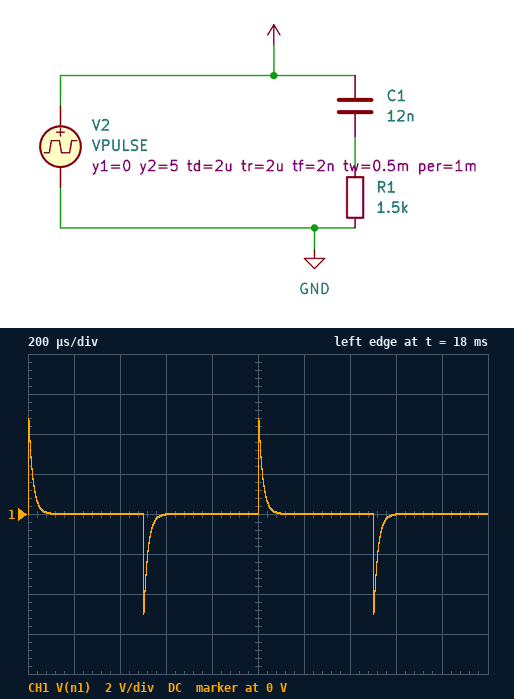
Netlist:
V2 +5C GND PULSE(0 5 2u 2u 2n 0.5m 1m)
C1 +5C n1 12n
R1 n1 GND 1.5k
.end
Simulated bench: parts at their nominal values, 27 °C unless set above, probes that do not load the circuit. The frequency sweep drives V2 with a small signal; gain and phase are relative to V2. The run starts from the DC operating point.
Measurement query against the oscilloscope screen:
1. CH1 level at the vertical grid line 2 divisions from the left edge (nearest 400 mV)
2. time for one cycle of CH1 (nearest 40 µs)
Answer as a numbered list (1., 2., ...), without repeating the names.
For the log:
1. 0 V
2. 1.00 ms
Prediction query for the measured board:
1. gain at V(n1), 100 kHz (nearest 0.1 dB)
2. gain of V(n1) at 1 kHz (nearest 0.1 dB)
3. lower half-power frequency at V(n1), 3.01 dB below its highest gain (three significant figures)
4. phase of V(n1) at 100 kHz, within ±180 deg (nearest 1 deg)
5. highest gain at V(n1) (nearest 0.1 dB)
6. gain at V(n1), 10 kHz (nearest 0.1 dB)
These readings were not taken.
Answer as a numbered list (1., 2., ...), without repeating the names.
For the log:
1. 0 dB
2. -19.0 dB
3. 8.84 kHz
4. 5 deg
5. 0 dB
6. -2.5 dB
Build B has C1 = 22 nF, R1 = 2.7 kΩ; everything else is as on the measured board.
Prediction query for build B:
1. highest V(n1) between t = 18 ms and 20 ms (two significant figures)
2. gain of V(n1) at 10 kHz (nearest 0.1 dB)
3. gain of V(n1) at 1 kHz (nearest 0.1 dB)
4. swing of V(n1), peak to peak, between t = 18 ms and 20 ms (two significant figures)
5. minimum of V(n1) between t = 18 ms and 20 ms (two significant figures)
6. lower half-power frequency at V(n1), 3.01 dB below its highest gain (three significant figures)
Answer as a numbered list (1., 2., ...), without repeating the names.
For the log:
1. 4.9 V
2. -0.3 dB
3. -9.1 dB
4. 9.9 V
5. -5.0 V
6. 2.68 kHz
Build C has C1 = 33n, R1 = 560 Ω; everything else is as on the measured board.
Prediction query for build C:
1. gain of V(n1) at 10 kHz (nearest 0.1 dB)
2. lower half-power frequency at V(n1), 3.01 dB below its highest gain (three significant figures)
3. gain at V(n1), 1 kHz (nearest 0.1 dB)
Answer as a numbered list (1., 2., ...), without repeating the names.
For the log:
1. -2.4 dB
2. 8.61 kHz
3. -18.8 dB
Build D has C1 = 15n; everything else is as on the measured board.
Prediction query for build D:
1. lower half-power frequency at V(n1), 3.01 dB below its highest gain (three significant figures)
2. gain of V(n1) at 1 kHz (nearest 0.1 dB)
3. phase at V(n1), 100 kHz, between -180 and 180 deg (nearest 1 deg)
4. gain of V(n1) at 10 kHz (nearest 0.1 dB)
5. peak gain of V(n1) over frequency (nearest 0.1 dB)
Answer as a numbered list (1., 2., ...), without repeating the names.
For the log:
1. 7.07 kHz
2. -17.1 dB
3. 4 deg
4. -1.8 dB
5. 0 dB
